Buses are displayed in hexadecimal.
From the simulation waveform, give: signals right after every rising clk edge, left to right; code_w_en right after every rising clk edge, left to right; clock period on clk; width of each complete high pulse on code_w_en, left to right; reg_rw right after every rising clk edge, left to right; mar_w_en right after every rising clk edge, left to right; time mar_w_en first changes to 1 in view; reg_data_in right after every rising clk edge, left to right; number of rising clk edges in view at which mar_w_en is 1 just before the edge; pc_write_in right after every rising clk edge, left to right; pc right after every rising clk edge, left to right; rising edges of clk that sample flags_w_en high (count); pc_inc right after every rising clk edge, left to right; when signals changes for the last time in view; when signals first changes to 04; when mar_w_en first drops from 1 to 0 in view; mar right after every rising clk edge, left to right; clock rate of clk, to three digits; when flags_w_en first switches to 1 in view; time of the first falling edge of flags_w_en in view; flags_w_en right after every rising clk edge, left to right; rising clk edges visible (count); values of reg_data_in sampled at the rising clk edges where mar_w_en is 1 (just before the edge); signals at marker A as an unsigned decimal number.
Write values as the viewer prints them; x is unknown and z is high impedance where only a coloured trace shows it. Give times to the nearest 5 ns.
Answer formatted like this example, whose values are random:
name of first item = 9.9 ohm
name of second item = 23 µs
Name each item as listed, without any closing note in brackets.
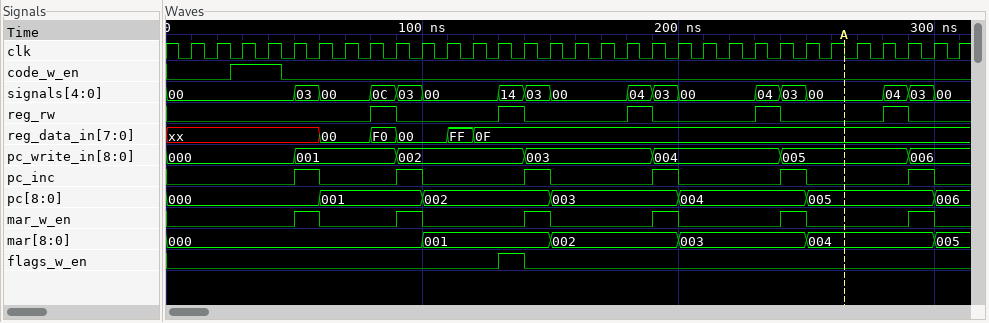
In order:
signals right after every rising clk edge, left to right = 00, 00, 00, 00, 03, 00, 00, 0C, 03, 00, 00, 00, 14, 03, 00, 00, 00, 04, 03, 00, 00, 00, 04, 03, 00, 00, 00, 04, 03, 00, 00
code_w_en right after every rising clk edge, left to right = 0 0 1 1 0 0 0 0 0 0 0 0 0 0 0 0 0 0 0 0 0 0 0 0 0 0 0 0 0 0 0
clock period on clk = 10 ns
width of each complete high pulse on code_w_en, left to right = 20 ns
reg_rw right after every rising clk edge, left to right = 0 0 0 0 0 0 0 1 0 0 0 0 1 0 0 0 0 1 0 0 0 0 1 0 0 0 0 1 0 0 0
mar_w_en right after every rising clk edge, left to right = 0 0 0 0 1 0 0 0 1 0 0 0 0 1 0 0 0 0 1 0 0 0 0 1 0 0 0 0 1 0 0
time mar_w_en first changes to 1 in view = 50 ns
reg_data_in right after every rising clk edge, left to right = xx, xx, xx, xx, xx, 00, 00, F0, 00, 00, FF, 0F, 0F, 0F, 0F, 0F, 0F, 0F, 0F, 0F, 0F, 0F, 0F, 0F, 0F, 0F, 0F, 0F, 0F, 0F, 0F
number of rising clk edges in view at which mar_w_en is 1 just before the edge = 6
pc_write_in right after every rising clk edge, left to right = 000, 000, 000, 000, 001, 001, 001, 001, 002, 002, 002, 002, 002, 003, 003, 003, 003, 003, 004, 004, 004, 004, 004, 005, 005, 005, 005, 005, 006, 006, 006
pc right after every rising clk edge, left to right = 000, 000, 000, 000, 000, 001, 001, 001, 001, 002, 002, 002, 002, 002, 003, 003, 003, 003, 003, 004, 004, 004, 004, 004, 005, 005, 005, 005, 005, 006, 006
rising edges of clk that sample flags_w_en high = 1
pc_inc right after every rising clk edge, left to right = 0 0 0 0 1 0 0 0 1 0 0 0 0 1 0 0 0 0 1 0 0 0 0 1 0 0 0 0 1 0 0
when signals changes for the last time in view = 300 ns
when signals first changes to 04 = 180 ns
when mar_w_en first drops from 1 to 0 in view = 60 ns
mar right after every rising clk edge, left to right = 000, 000, 000, 000, 000, 000, 000, 000, 000, 001, 001, 001, 001, 001, 002, 002, 002, 002, 002, 003, 003, 003, 003, 003, 004, 004, 004, 004, 004, 005, 005
clock rate of clk, to three digits = 100 MHz
when flags_w_en first switches to 1 in view = 130 ns
time of the first falling edge of flags_w_en in view = 140 ns
flags_w_en right after every rising clk edge, left to right = 0 0 0 0 0 0 0 0 0 0 0 0 1 0 0 0 0 0 0 0 0 0 0 0 0 0 0 0 0 0 0
rising clk edges visible = 31
values of reg_data_in sampled at the rising clk edges where mar_w_en is 1 = xx, 00, 0F, 0F, 0F, 0F
signals at marker A as an unsigned decimal number = 0
